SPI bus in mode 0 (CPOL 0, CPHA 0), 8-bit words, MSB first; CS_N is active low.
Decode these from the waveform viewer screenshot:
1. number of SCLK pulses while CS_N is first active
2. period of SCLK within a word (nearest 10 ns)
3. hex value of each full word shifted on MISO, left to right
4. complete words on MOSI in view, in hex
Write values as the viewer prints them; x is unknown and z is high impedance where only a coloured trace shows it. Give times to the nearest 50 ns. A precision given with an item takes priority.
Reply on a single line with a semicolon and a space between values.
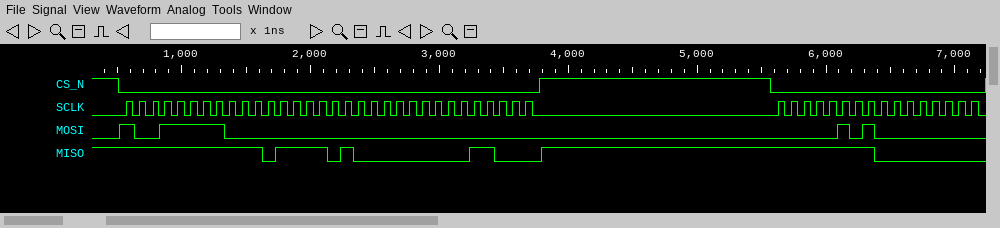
32; 100 ns; FF, EF, 40, 18, FF, 00; 9F, 00, 00, 00, 05, 00
